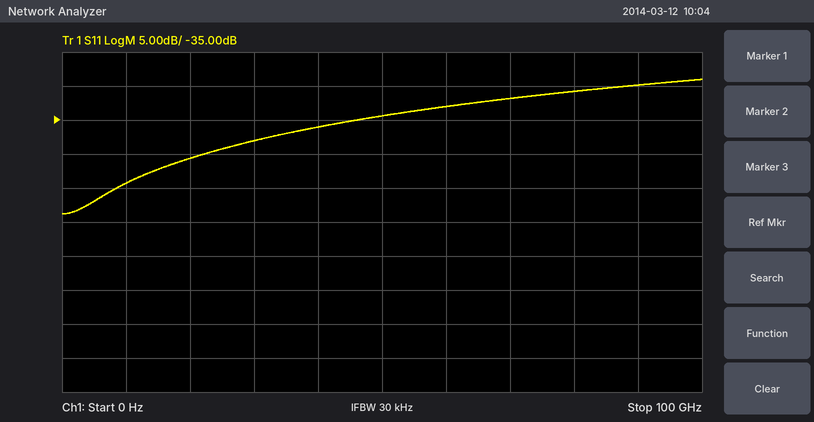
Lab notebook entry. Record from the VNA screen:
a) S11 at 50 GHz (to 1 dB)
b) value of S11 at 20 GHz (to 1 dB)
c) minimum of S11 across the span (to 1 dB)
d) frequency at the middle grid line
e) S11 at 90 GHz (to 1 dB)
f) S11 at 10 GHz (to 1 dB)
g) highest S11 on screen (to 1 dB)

-34 dB
-41 dB
-49 dB
50 GHz
-30 dB
-44 dB
-29 dB
